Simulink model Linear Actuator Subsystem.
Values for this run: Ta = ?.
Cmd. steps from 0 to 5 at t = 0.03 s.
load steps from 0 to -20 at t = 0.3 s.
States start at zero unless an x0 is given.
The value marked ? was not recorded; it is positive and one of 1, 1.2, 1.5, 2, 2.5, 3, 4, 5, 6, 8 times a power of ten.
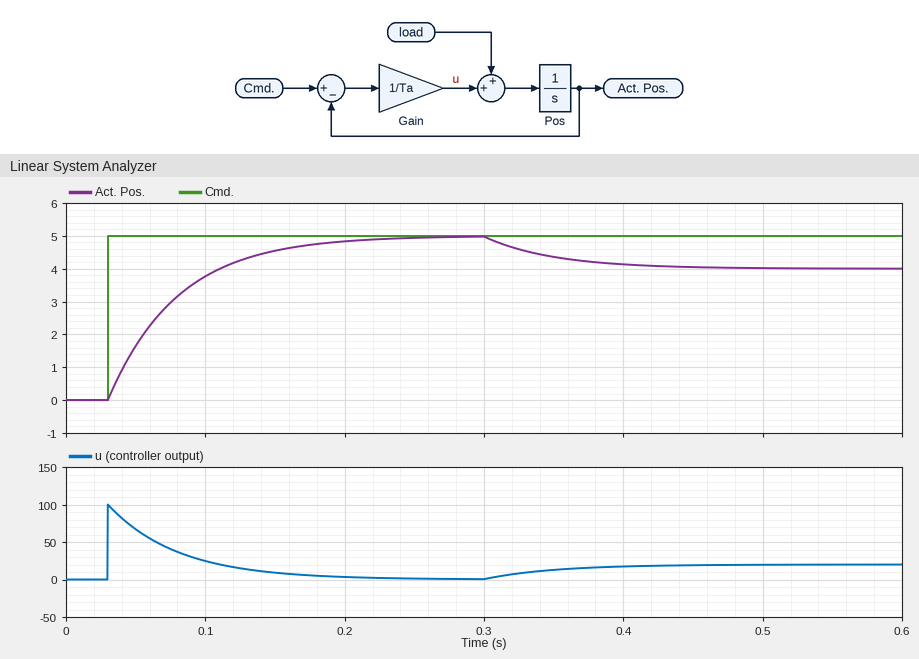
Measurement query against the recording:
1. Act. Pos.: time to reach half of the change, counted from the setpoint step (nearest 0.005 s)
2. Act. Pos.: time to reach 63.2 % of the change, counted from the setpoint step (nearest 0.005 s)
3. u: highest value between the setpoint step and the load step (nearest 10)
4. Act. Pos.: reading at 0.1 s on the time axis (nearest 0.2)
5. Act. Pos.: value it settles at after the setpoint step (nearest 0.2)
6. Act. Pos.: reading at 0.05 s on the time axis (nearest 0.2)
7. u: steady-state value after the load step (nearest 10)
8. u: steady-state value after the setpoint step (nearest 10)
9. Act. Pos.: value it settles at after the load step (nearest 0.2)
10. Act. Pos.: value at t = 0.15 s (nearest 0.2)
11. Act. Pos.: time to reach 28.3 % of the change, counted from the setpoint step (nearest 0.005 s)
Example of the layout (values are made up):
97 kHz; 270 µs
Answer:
0.035 s; 0.050 s; 100; 3.8; 5.0; 1.6; 20; 0; 4.0; 4.6; 0.015 s
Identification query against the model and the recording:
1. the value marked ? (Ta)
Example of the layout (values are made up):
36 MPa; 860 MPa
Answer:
0.05
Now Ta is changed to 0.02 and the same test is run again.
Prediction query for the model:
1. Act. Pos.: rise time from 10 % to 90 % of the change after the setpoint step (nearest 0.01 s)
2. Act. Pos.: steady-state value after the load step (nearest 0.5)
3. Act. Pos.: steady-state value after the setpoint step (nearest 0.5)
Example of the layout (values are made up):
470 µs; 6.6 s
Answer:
0.04 s; 4.5; 5.0
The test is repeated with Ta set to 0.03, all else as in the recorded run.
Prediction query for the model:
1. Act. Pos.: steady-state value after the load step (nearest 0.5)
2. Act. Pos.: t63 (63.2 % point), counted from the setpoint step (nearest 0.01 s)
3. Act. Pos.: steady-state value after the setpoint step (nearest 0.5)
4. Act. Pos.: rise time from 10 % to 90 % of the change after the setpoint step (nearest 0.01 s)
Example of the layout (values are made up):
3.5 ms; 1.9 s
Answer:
4.5; 0.03 s; 5.0; 0.07 s
